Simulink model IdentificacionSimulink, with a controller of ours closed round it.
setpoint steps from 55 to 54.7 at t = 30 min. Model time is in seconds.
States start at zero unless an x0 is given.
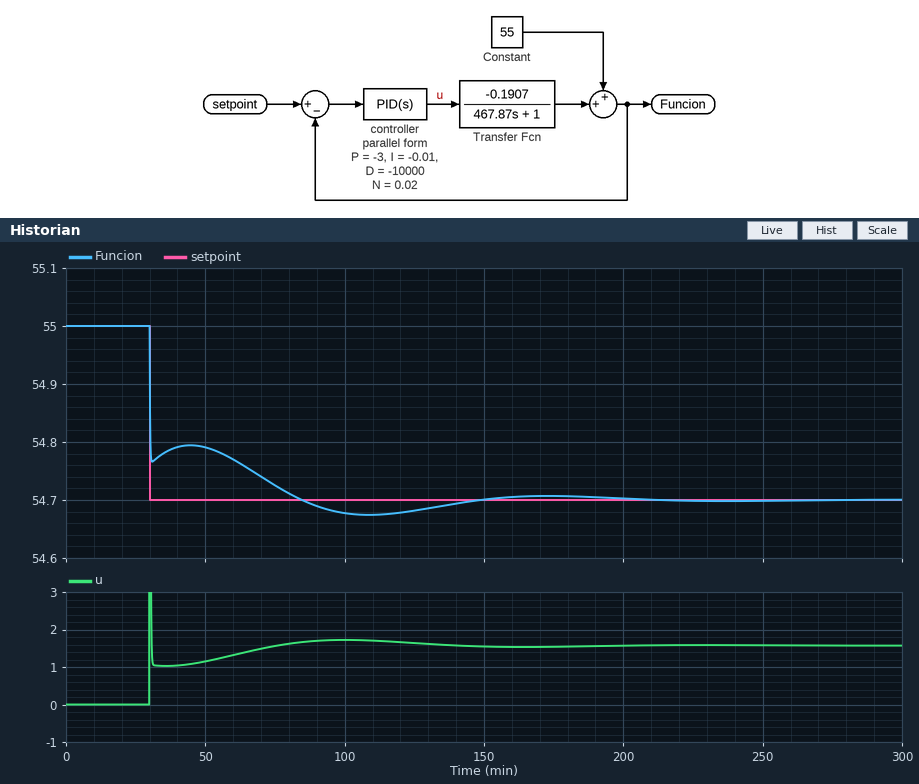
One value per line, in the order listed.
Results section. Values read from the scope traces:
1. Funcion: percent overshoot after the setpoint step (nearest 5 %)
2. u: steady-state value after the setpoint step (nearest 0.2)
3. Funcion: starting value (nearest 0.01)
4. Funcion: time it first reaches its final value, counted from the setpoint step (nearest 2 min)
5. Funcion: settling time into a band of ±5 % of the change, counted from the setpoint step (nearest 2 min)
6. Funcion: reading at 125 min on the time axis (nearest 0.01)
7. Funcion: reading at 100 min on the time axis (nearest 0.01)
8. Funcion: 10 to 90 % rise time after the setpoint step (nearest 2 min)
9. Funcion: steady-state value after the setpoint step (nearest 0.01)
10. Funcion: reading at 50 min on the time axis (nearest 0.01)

10 %
1.6
55.00
54 min
100 min
54.68
54.68
44 min
54.70
54.79
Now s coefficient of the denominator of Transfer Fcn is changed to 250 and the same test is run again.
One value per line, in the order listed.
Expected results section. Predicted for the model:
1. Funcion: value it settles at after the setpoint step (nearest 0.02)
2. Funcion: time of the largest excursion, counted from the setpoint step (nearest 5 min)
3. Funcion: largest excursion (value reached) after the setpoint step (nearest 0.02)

54.70
80 min
54.68
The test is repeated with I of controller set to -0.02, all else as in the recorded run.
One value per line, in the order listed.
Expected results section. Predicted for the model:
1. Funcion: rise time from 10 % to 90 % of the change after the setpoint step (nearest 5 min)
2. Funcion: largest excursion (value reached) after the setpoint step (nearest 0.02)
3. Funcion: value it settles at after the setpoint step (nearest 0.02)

25 min
54.66
54.70
